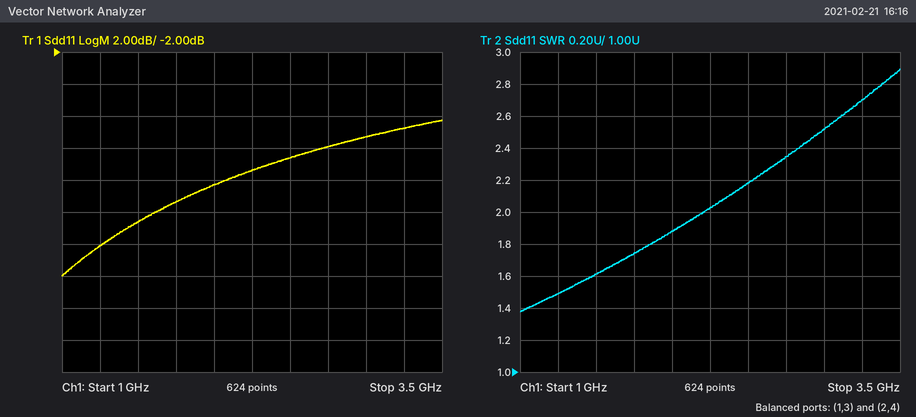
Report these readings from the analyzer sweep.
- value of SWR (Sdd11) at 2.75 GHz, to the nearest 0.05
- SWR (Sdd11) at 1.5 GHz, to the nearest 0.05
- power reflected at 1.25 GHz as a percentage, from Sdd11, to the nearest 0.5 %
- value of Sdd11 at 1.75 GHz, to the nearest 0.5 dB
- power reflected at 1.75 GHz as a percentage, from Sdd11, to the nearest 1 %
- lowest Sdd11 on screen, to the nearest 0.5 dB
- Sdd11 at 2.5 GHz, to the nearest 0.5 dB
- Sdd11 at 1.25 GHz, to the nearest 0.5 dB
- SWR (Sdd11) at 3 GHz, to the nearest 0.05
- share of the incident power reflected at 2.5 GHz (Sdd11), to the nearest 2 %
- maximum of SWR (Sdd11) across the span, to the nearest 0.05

2.35
1.60
4.0 %
-11.5 dB
7 %
-16.0 dB
-8.5 dB
-14.0 dB
2.50
14 %
2.90
